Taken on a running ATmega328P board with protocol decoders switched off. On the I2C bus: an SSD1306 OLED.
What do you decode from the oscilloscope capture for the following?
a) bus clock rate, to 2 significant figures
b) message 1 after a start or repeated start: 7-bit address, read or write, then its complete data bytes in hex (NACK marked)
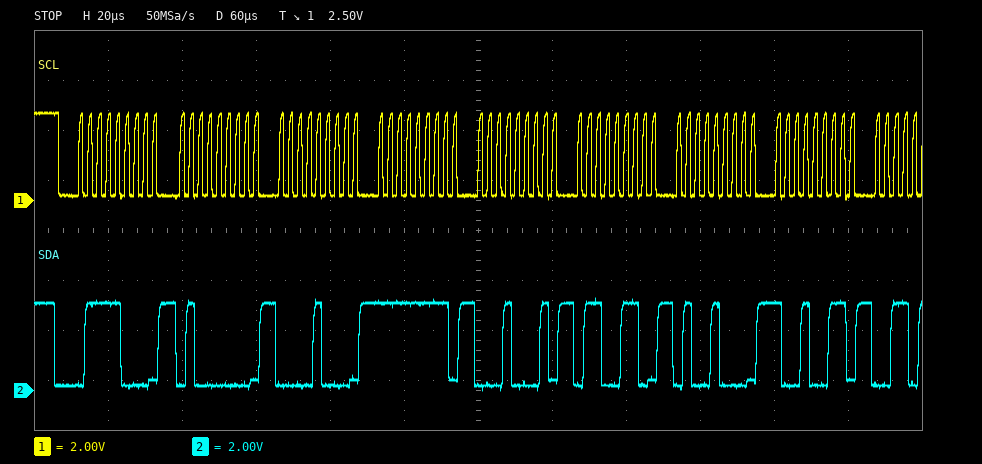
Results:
400 kHz
0x3C write: 40 08 FF 11 66 48 93
